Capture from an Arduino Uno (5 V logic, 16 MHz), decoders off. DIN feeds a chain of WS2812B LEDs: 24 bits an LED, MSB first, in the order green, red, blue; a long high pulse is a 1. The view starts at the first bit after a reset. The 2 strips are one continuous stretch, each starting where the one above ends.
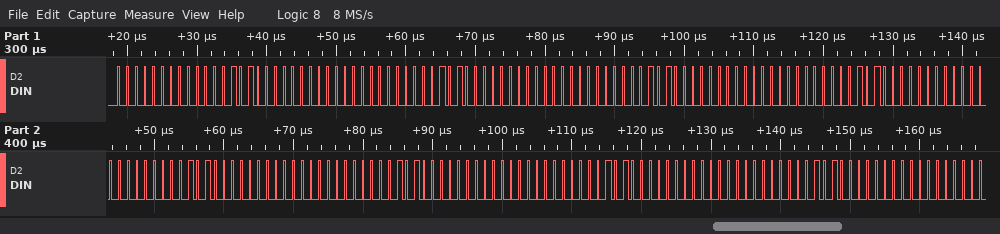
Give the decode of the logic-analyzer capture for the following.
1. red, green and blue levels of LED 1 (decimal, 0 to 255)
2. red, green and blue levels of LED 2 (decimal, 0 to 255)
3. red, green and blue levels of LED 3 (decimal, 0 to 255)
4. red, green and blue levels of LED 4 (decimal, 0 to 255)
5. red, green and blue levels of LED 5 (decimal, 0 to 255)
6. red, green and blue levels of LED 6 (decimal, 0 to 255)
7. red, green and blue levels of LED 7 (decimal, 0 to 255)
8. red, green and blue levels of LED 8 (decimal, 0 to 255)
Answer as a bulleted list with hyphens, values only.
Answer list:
- 5, 0, 0
- 5, 0, 0
- 5, 0, 0
- 5, 0, 0
- 5, 0, 0
- 5, 0, 0
- 5, 0, 0
- 5, 0, 0
